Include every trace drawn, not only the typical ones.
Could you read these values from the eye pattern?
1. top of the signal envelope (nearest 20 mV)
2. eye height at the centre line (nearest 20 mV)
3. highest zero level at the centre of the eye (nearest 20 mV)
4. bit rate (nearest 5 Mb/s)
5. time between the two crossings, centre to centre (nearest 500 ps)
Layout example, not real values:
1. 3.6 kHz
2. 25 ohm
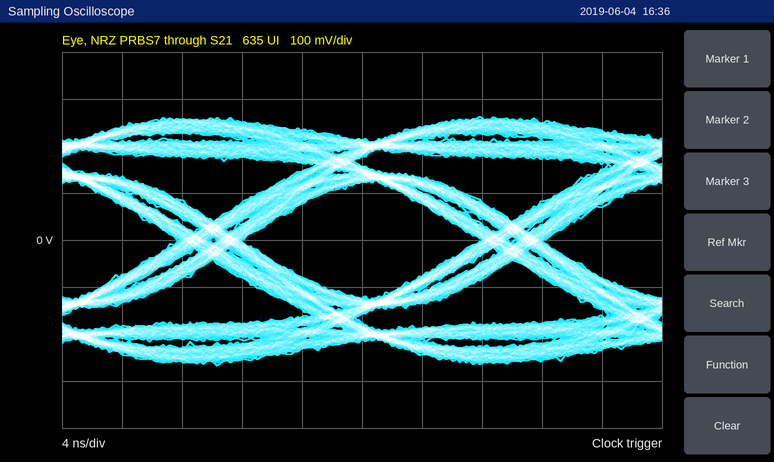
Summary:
1. 260 mV
2. 240 mV
3. -120 mV
4. 50 Mb/s
5. 20.0 ns
